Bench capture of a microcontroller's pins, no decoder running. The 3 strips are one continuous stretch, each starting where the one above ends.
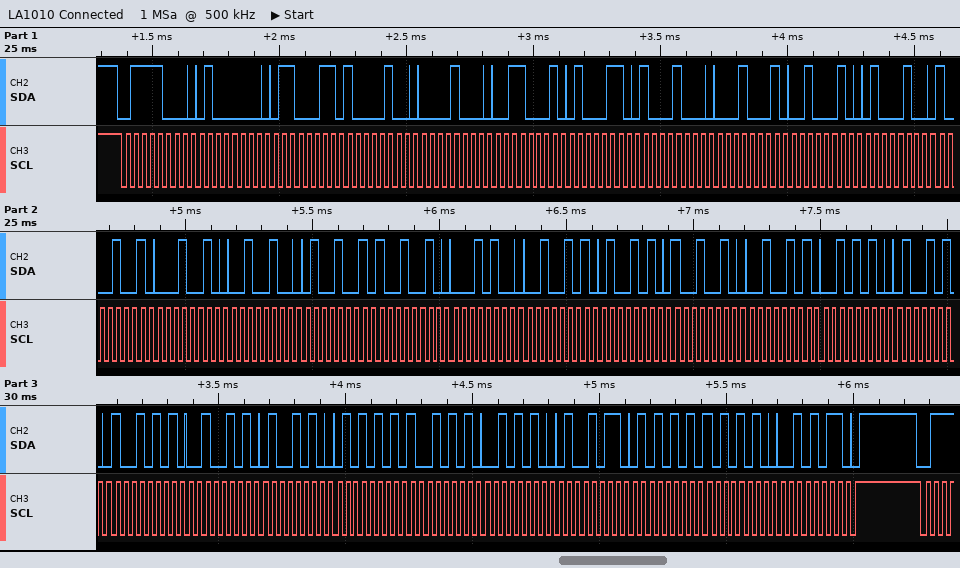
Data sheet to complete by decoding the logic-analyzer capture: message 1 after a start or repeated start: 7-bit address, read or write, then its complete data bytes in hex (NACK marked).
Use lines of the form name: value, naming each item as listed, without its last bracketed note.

message 1 after a start or repeated start: 7-bit address, read or write, then its complete data bytes in hex: 0x3C write: 40 63 84 08 31 46 88 11 22 44 89 12 24 49 92 14 25 4A 92 25 2A 4A 95 25 4A 55 95 2A 4B 55 AA 2B
